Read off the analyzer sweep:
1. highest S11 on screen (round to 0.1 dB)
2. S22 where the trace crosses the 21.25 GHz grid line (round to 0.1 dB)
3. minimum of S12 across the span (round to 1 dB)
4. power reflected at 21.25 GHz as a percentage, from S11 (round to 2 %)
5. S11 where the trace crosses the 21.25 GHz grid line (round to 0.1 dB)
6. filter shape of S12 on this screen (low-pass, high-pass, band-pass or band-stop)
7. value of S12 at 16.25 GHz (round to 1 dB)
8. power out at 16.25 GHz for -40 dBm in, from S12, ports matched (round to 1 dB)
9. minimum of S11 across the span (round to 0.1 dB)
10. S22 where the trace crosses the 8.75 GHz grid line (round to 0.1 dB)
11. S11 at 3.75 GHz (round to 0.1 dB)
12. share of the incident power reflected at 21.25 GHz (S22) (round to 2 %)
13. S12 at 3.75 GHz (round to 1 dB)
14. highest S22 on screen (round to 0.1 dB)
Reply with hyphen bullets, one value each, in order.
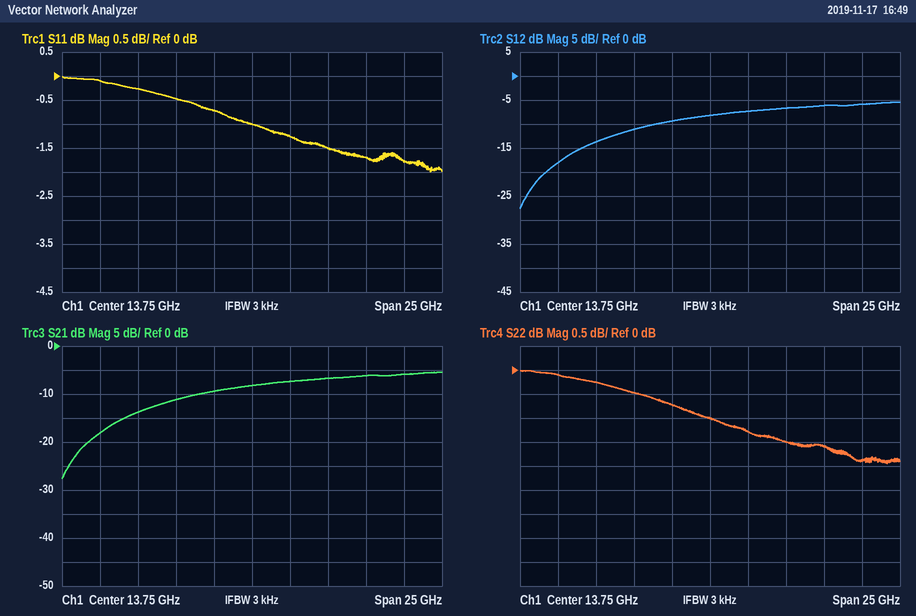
- 0.0 dB
- -1.6 dB
- -28 dB
- 68 %
- -1.7 dB
- high-pass
- -7 dB
- -47 dBm
- -2.0 dB
- -0.5 dB
- -0.1 dB
- 70 %
- -18 dB
- 0.0 dB
